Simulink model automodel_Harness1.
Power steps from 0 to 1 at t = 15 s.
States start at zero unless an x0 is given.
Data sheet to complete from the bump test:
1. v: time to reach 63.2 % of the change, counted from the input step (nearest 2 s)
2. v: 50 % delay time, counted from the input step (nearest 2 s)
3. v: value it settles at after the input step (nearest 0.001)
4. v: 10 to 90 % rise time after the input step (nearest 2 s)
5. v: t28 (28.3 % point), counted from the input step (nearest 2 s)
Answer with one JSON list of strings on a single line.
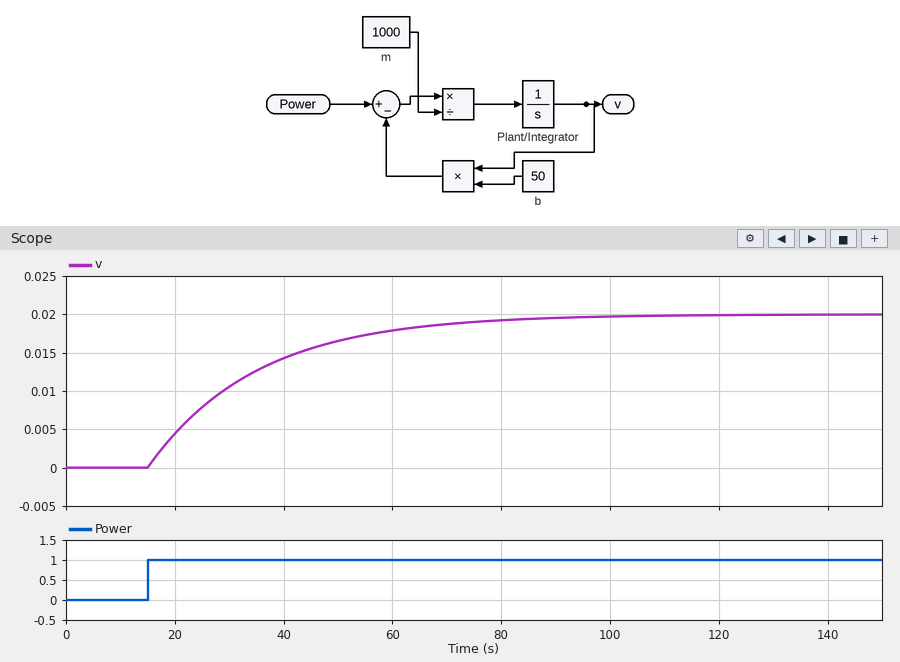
["20 s", "14 s", "0.020", "44 s", "6 s"]
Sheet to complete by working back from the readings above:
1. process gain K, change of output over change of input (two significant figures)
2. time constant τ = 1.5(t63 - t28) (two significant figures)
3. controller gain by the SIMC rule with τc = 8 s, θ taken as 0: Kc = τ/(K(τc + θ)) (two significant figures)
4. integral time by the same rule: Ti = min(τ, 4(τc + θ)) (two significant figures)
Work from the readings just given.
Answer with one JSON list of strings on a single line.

["0.020", "21 s", "130", "21 s"]
